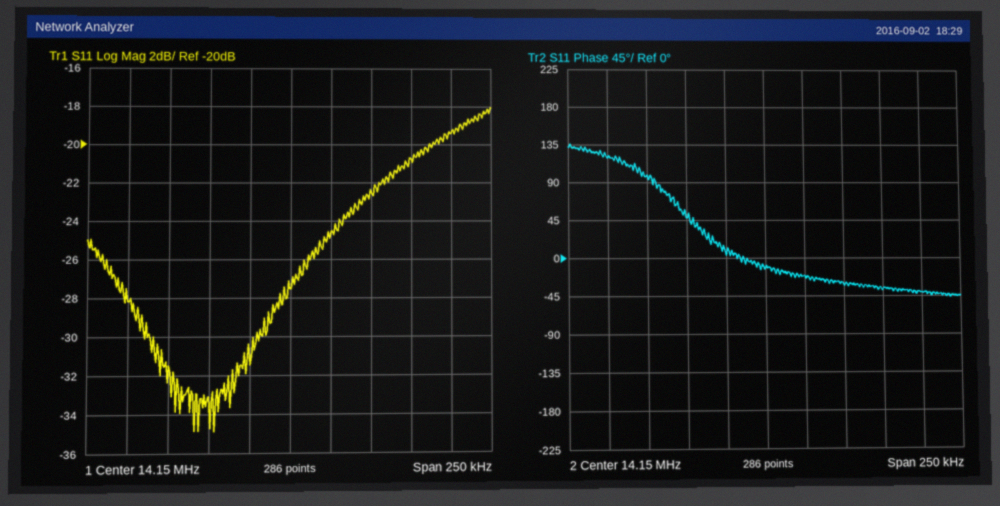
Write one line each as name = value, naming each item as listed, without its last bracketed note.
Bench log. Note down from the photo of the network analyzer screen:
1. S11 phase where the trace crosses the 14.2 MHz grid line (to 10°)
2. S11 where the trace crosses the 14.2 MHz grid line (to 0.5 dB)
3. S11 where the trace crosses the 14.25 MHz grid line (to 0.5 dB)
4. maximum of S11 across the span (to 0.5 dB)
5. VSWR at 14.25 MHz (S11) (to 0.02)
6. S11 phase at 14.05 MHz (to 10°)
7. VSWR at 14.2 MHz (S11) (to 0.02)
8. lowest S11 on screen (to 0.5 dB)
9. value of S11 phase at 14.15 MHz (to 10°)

S11 phase where the trace crosses the 14.2 MHz grid line = -30°
S11 where the trace crosses the 14.2 MHz grid line = -22.5 dB
S11 where the trace crosses the 14.25 MHz grid line = -19.5 dB
maximum of S11 across the span = -18.0 dB
VSWR at 14.25 MHz (S11) = 1.24
S11 phase at 14.05 MHz = 120°
VSWR at 14.2 MHz (S11) = 1.16
lowest S11 on screen = -35.0 dB
value of S11 phase at 14.15 MHz = -10°
